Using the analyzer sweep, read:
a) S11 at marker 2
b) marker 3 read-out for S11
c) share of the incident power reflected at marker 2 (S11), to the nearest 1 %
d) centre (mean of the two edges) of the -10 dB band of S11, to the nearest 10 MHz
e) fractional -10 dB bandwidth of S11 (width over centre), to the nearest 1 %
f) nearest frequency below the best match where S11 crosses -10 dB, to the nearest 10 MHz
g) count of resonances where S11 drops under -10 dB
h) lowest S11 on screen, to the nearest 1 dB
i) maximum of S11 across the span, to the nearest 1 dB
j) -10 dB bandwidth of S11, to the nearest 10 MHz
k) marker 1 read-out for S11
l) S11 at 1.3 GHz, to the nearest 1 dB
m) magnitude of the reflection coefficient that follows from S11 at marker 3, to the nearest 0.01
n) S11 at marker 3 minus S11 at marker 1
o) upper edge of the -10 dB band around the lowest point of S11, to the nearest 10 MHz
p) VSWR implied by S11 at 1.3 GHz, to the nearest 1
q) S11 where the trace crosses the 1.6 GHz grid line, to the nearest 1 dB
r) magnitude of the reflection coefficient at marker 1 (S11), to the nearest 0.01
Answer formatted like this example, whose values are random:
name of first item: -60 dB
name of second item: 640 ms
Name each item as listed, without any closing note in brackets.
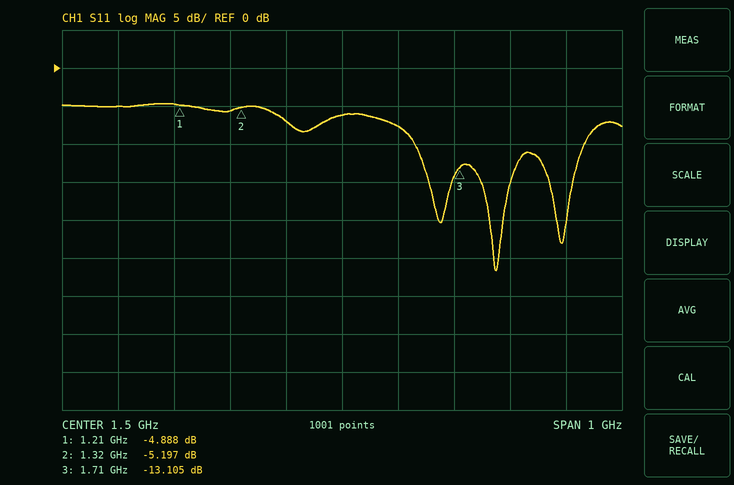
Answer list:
S11 at marker 2: -5.197 dB
marker 3 read-out for S11: -13.105 dB
share of the incident power reflected at marker 2 (S11), to the nearest 1 %: 30 %
centre (mean of the two edges) of the -10 dB band of S11, to the nearest 10 MHz: 1.78 GHz
fractional -10 dB bandwidth of S11 (width over centre), to the nearest 1 %: 17 %
nearest frequency below the best match where S11 crosses -10 dB, to the nearest 10 MHz: 1.63 GHz
count of resonances where S11 drops under -10 dB: 3
lowest S11 on screen, to the nearest 1 dB: -27 dB
maximum of S11 across the span, to the nearest 1 dB: -5 dB
-10 dB bandwidth of S11, to the nearest 10 MHz: 300 MHz
marker 1 read-out for S11: -4.888 dB
S11 at 1.3 GHz, to the nearest 1 dB: -6 dB
magnitude of the reflection coefficient that follows from S11 at marker 3, to the nearest 0.01: 0.22
S11 at marker 3 minus S11 at marker 1: -8.217 dB
upper edge of the -10 dB band around the lowest point of S11, to the nearest 10 MHz: 1.93 GHz
VSWR implied by S11 at 1.3 GHz, to the nearest 1: 3
S11 where the trace crosses the 1.6 GHz grid line, to the nearest 1 dB: -8 dB
magnitude of the reflection coefficient at marker 1 (S11), to the nearest 0.01: 0.57
